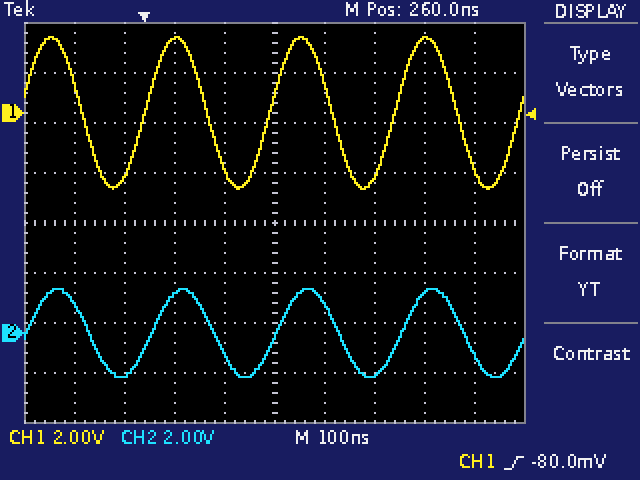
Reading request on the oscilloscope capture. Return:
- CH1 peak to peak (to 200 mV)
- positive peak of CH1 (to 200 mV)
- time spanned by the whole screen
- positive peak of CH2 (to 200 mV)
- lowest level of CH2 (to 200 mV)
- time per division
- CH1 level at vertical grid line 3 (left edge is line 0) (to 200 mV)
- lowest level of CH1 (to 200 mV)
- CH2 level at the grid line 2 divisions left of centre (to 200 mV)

6.0 V
3.0 V
1 µs
1.8 V
-1.8 V
100 ns
3.0 V
-3.0 V
1.6 V
